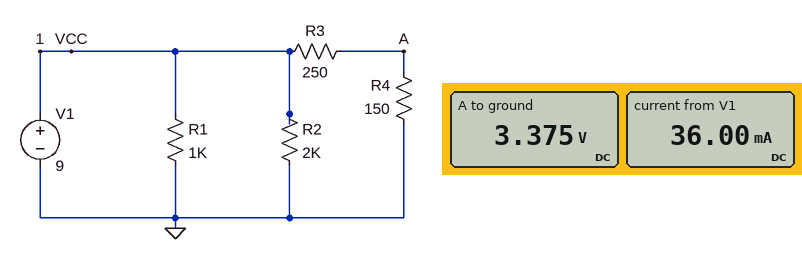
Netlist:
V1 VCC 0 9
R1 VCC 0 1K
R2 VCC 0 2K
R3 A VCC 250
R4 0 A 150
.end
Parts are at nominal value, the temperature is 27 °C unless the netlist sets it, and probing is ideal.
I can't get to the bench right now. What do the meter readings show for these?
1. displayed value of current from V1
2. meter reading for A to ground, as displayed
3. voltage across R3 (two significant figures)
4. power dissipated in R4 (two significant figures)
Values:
36.00 mA
3.375 V
5.6 V
76 mW
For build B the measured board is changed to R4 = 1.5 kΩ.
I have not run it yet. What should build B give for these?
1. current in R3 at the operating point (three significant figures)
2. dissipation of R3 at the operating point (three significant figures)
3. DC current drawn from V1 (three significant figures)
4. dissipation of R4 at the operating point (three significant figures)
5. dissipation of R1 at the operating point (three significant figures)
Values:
5.14 mA
6.61 mW
18.6 mA
39.7 mW
81.0 mW
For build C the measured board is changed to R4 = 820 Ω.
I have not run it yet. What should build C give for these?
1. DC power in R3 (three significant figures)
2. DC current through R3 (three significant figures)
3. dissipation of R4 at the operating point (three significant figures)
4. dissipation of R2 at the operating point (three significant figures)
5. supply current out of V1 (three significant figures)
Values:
17.7 mW
8.41 mA
58.0 mW
40.5 mW
21.9 mA
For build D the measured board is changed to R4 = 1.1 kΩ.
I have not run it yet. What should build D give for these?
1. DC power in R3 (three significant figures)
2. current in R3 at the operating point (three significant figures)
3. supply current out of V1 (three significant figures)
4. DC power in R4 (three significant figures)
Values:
11.1 mW
6.67 mA
20.2 mA
48.9 mW
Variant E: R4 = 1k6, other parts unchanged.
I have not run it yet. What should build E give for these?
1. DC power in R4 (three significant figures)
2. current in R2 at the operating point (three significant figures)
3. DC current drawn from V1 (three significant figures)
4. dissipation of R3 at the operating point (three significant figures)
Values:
37.9 mW
4.50 mA
18.4 mA
5.92 mW
